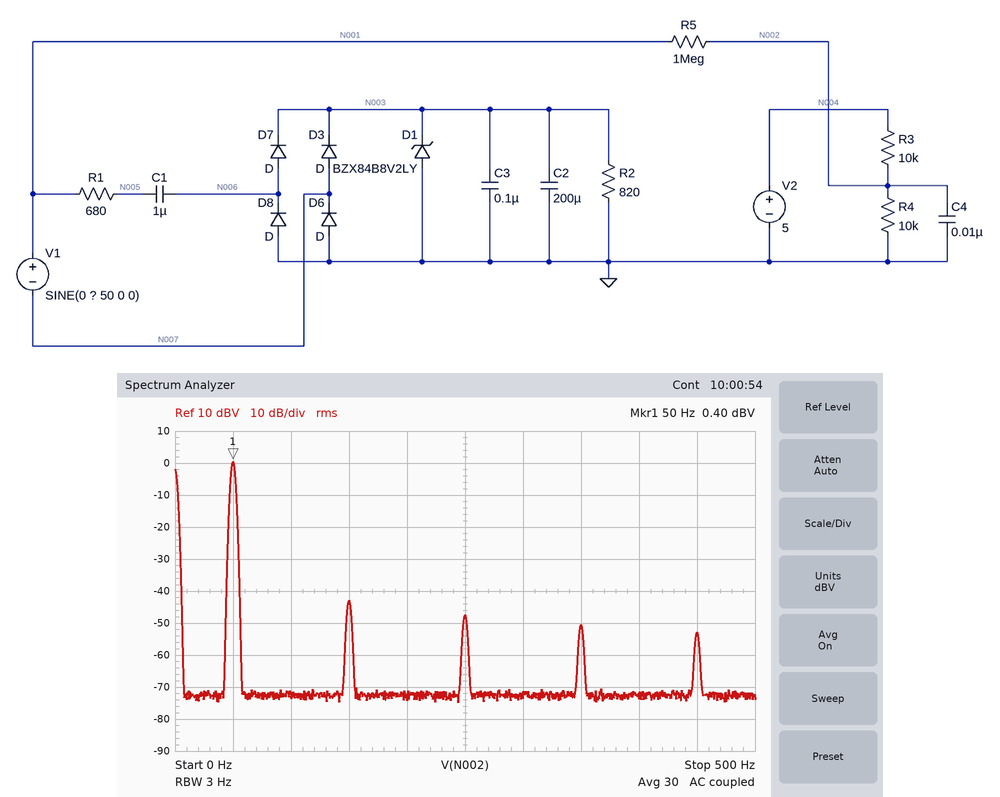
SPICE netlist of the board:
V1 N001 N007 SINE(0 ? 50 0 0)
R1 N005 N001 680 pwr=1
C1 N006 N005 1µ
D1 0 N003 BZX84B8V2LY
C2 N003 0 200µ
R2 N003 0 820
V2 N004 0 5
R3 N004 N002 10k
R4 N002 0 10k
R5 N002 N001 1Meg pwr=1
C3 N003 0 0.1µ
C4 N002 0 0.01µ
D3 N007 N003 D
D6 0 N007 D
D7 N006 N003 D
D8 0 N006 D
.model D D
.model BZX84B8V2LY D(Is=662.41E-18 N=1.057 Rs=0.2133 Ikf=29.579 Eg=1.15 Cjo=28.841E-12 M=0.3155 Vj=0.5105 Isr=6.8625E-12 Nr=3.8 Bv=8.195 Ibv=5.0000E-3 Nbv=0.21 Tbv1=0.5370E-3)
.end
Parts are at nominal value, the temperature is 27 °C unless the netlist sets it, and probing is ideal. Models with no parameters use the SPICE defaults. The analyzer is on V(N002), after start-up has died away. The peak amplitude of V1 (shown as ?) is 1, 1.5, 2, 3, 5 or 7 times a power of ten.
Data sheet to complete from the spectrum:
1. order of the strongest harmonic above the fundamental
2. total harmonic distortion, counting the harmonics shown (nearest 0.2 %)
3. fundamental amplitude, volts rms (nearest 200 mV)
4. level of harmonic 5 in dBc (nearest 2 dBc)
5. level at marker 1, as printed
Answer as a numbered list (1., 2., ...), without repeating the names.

1. 3
2. 0.8 %
3. 1.0 V
4. -48 dBc
5. 0.40 dBV
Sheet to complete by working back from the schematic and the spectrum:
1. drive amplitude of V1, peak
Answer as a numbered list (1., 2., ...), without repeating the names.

1. 300 V
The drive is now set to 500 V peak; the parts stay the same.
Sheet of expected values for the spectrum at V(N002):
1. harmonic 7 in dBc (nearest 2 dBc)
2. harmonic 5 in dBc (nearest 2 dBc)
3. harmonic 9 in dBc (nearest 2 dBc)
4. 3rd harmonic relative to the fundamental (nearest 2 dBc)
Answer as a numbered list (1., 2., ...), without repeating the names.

1. -56 dBc
2. -52 dBc
3. -58 dBc
4. -48 dBc
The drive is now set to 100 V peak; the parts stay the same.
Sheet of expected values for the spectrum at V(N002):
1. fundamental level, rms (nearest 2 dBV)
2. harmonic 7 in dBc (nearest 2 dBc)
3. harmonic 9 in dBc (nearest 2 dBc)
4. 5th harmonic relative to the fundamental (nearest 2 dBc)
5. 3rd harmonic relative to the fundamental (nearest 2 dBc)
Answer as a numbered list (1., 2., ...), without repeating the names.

1. -10 dBV
2. -42 dBc
3. -44 dBc
4. -38 dBc
5. -34 dBc
